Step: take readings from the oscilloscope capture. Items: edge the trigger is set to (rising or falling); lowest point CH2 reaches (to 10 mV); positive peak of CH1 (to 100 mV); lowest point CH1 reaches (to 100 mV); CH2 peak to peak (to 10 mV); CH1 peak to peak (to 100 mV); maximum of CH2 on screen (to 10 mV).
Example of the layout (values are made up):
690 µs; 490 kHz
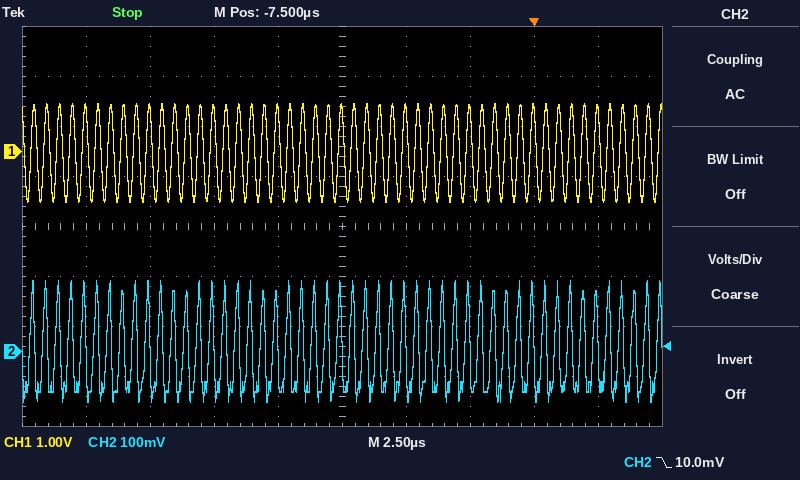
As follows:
falling; -100 mV; 1.0 V; -1.0 V; 240 mV; 2.0 V; 140 mV
